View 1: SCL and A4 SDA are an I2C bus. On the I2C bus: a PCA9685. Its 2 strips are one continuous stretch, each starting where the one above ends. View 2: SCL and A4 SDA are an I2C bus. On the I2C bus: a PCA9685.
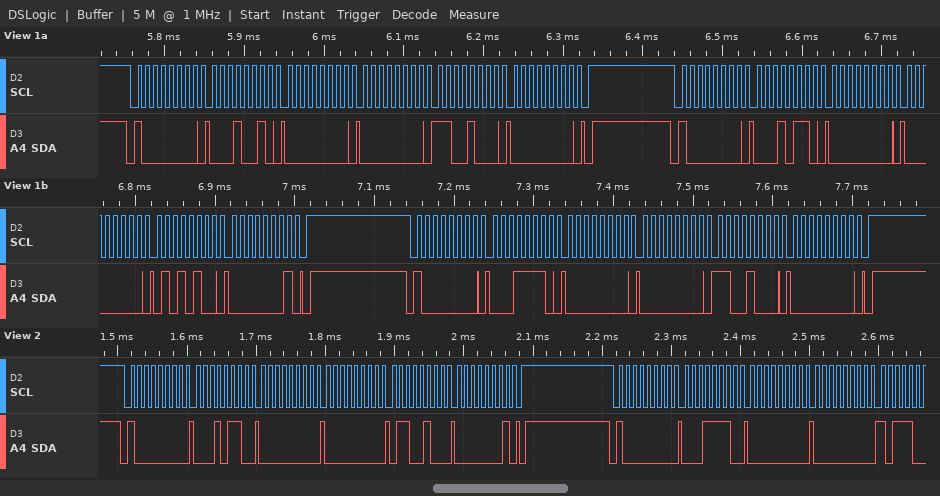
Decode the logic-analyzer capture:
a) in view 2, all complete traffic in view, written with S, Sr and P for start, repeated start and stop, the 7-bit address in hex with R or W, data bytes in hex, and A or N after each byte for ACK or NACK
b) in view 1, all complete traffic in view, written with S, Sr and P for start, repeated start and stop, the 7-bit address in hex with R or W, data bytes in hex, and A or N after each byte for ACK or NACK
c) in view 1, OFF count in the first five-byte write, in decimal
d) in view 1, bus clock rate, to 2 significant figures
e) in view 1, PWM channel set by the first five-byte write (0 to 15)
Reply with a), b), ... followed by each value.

a) S 40W A 16 A 00 A 00 A 64 A 01 A P S 40W A 1E A 00 A 00 A
b) S 40W A 12 A 00 A 00 A C8 A 00 A P S 40W A 16 A 00 A 00 A 54 A 01 A P S 40W A 1E A 00 A 00 A C8 A 00 A P
c) 200
d) 100 kHz
e) 3
